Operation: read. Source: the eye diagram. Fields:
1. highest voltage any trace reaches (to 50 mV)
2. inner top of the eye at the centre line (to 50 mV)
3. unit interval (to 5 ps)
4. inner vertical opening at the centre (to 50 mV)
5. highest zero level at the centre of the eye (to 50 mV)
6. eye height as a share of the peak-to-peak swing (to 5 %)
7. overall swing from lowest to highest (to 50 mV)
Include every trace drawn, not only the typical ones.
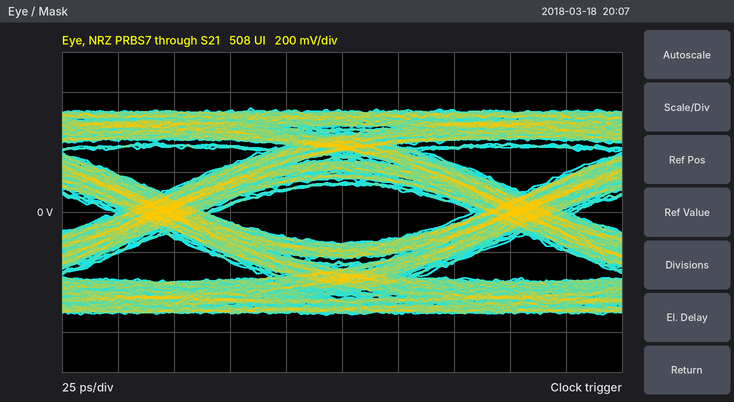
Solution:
500 mV
150 mV
160 ps
300 mV
-150 mV
30 %
1.05 V
